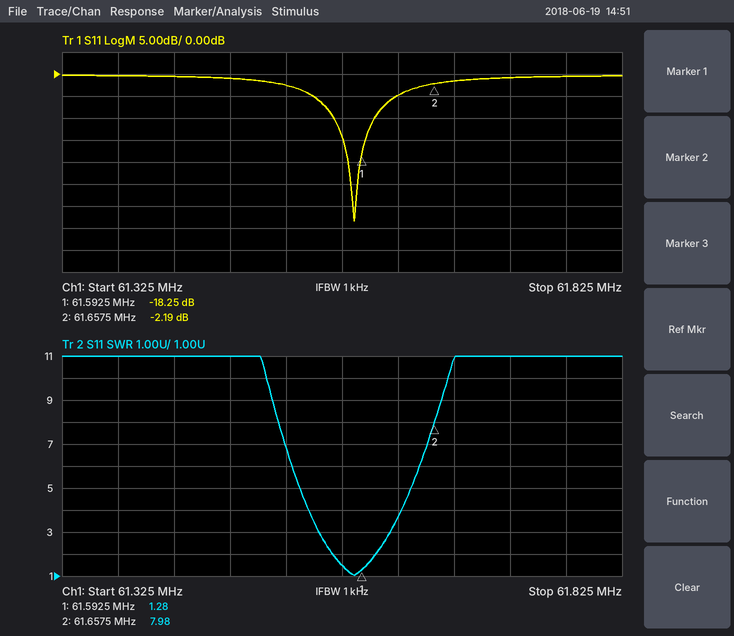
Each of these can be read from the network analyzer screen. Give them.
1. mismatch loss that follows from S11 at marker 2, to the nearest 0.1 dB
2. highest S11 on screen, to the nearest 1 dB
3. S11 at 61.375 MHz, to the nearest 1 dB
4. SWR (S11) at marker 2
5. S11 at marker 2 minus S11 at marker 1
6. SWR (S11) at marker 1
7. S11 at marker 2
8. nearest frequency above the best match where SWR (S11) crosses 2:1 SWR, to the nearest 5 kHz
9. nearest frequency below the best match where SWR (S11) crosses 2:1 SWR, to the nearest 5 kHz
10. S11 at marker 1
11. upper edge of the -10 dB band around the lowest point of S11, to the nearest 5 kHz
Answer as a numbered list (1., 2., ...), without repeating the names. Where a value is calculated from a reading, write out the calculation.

1. −10 log10(1 − 10^(-2.19/10)) ≈ 4.0 dB
2. 0 dB
3. 0 dB
4. 7.98
5. -2.19 − (-18.25) = 16.06 dB
6. 1.28
7. -2.19 dB
8. 61.605 MHz
9. 61.565 MHz
10. -18.25 dB
11. 61.605 MHz
